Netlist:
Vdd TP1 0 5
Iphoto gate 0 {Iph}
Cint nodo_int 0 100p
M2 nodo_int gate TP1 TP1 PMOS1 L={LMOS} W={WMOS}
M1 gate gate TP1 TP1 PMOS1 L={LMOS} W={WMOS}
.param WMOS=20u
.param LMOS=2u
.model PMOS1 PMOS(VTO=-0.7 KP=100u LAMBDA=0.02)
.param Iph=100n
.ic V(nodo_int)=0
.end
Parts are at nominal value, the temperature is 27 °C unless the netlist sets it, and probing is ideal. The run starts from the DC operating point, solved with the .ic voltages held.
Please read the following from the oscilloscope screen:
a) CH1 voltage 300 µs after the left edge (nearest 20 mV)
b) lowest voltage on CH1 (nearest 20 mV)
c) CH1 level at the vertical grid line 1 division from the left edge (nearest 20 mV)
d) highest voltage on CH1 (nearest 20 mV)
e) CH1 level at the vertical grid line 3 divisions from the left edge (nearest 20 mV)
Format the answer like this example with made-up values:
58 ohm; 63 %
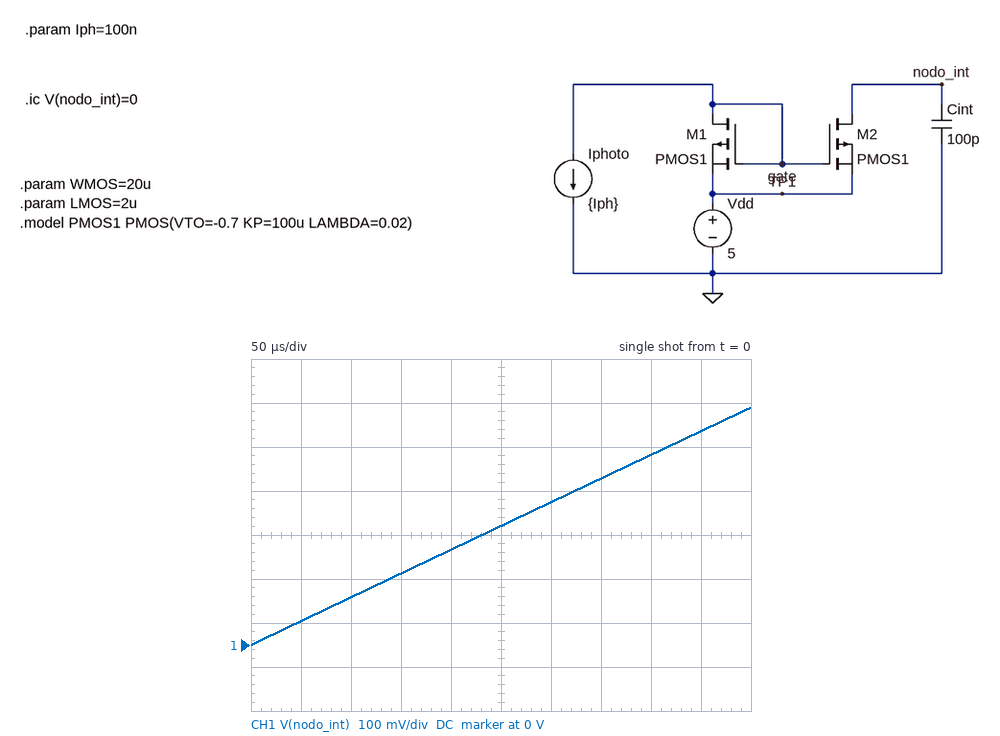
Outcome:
320 mV; 0 V; 60 mV; 540 mV; 160 mV
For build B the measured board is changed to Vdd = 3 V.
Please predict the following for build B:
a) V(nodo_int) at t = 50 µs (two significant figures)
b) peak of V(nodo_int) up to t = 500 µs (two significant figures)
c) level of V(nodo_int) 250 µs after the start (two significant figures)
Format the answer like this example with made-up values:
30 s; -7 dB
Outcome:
52 mV; 520 mV; 260 mV
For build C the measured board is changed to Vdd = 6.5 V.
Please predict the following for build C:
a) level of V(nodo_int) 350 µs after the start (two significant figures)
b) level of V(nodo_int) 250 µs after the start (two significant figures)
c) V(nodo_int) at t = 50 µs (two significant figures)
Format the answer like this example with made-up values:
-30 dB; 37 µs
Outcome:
390 mV; 280 mV; 56 mV
